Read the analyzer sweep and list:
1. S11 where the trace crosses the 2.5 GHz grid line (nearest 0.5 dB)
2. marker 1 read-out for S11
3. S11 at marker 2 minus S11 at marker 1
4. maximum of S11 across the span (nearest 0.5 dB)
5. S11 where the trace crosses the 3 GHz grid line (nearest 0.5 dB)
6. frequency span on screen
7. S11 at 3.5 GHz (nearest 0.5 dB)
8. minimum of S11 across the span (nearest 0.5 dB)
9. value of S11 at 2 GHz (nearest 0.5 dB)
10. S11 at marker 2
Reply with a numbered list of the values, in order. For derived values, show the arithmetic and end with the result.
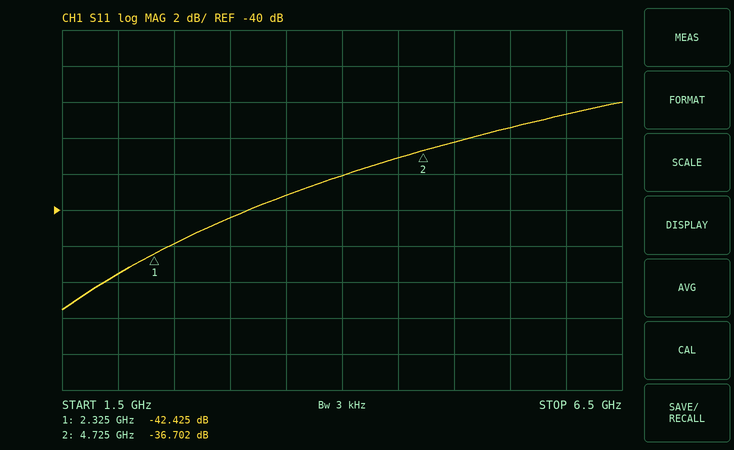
1. -42.0 dB
2. -42.425 dB
3. -36.702 − (-42.425) = 5.723 dB
4. -34.0 dB
5. -40.5 dB
6. 5 GHz
7. -39.0 dB
8. -45.5 dB
9. -43.5 dB
10. -36.702 dB
